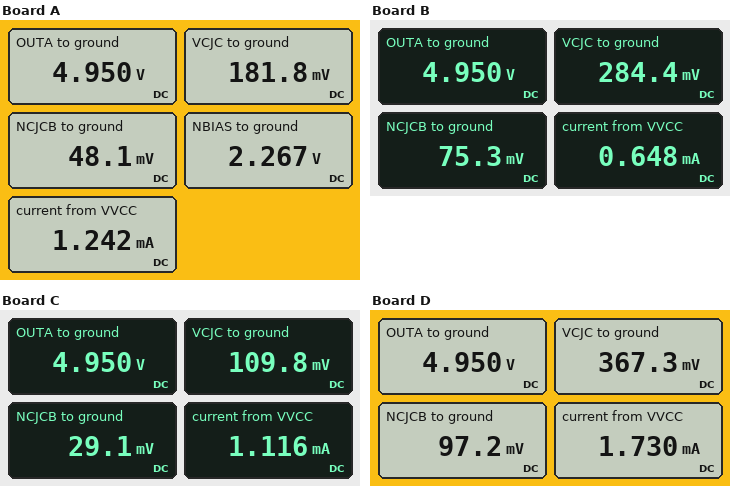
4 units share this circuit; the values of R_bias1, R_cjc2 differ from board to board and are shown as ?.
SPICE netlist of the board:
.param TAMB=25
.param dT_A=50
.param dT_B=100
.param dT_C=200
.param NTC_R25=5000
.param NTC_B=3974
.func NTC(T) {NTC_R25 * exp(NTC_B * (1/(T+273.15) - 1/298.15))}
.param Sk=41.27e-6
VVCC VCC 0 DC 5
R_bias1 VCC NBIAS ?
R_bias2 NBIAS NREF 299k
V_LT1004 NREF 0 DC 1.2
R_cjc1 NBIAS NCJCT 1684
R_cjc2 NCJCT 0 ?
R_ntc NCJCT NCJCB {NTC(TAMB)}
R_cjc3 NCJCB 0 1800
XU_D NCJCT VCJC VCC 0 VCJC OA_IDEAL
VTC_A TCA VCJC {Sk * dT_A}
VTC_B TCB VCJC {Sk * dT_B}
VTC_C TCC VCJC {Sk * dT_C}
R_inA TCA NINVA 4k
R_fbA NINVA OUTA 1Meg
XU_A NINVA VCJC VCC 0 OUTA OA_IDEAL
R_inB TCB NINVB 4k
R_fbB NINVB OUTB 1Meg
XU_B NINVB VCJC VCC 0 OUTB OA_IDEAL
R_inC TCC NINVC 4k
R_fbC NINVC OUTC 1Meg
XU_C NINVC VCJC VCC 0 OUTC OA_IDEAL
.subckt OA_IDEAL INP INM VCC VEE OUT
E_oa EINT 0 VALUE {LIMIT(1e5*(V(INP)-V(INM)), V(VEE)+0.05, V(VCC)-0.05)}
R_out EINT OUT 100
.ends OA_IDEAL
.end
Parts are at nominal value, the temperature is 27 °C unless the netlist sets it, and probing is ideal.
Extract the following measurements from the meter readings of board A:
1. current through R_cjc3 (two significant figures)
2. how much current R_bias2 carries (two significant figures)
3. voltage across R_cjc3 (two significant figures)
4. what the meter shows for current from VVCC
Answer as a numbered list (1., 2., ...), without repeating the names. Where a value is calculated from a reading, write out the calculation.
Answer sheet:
1. (48.1 mV) / 1.8 kΩ = 27 µA
2. (2.267 V - 1.2 V) / 299 kΩ = 3.6 µA
3. 48.1 mV = 48 mV
4. 1.242 mA
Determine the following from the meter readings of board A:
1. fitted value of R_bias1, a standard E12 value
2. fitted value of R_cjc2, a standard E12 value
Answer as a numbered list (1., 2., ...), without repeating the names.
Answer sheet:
1. 2.2 kΩ
2. 150 Ω
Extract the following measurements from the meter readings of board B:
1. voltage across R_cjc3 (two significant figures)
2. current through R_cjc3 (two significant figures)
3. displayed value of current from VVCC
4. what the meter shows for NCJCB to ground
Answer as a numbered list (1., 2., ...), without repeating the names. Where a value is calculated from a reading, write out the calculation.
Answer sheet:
1. 75.3 mV = 75 mV
2. (75.3 mV) / 1.8 kΩ = 42 µA
3. 0.648 mA
4. 75.3 mV
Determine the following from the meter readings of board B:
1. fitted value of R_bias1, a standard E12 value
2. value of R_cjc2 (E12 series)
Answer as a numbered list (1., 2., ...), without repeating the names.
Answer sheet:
1. 5.6 kΩ
2. 470 Ω
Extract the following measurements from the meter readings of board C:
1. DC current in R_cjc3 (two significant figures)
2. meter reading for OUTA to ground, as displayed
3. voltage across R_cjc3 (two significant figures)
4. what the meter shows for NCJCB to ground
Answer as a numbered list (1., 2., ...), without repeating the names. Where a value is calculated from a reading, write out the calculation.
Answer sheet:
1. (29.1 mV) / 1.8 kΩ = 16 µA
2. 4.950 V
3. 29.1 mV = 29 mV
4. 29.1 mV
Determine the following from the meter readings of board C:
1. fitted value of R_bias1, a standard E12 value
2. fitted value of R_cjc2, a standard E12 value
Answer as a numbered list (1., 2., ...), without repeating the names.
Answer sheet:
1. 2.7 kΩ
2. 100 Ω
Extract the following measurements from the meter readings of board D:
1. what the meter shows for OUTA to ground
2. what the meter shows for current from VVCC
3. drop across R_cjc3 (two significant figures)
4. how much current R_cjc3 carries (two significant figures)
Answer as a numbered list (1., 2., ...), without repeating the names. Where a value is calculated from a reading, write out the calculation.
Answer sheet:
1. 4.950 V
2. 1.730 mA
3. 97.2 mV = 97 mV
4. (97.2 mV) / 1.8 kΩ = 54 µA
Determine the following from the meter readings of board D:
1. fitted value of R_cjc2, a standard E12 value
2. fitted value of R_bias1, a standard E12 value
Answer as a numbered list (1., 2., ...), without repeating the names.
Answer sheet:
1. 220 Ω
2. 1 kΩ
